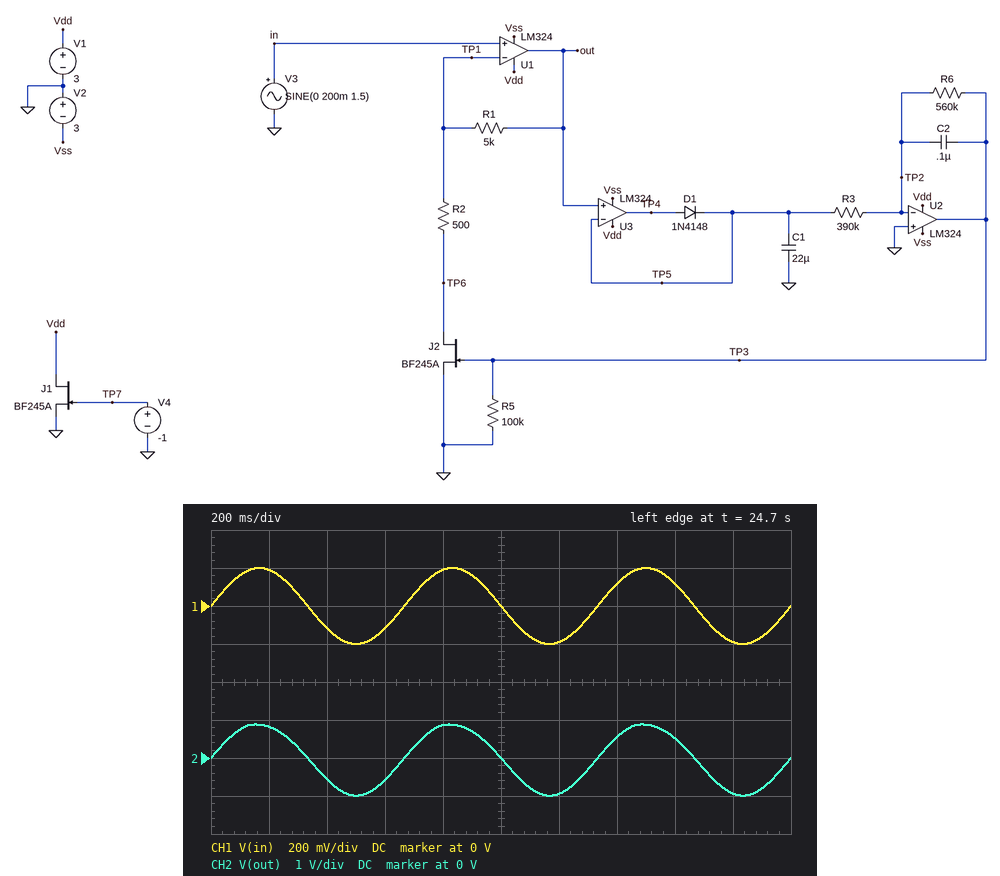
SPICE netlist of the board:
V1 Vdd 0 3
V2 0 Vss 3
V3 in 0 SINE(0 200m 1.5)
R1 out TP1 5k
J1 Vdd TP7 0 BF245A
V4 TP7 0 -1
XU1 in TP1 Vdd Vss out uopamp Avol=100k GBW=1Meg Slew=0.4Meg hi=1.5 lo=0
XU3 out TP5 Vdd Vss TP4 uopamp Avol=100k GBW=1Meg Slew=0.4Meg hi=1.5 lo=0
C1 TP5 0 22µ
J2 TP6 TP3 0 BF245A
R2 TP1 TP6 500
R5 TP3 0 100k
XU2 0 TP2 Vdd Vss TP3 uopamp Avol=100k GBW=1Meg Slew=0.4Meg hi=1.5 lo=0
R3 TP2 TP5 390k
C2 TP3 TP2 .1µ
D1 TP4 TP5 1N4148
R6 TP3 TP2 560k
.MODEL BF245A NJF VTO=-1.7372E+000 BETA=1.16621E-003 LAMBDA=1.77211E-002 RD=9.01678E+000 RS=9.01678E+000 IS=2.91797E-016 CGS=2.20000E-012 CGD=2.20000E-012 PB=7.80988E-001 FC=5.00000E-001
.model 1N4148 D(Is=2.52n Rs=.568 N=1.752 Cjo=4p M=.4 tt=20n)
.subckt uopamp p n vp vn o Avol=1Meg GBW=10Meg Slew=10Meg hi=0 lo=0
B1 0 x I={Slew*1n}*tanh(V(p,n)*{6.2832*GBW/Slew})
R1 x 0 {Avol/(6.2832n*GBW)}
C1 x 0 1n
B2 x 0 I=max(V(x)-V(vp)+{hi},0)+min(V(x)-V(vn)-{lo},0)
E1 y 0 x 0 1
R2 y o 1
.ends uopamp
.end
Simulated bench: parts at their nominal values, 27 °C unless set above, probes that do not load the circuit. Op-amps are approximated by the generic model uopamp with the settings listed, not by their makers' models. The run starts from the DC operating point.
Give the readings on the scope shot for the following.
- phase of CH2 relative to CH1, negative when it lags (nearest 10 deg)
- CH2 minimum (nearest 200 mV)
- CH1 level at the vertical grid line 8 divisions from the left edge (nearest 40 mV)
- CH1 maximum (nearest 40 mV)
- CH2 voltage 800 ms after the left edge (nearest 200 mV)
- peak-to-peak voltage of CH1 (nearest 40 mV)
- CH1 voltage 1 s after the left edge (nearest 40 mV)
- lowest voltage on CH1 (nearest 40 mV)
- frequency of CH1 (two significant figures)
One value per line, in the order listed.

0 deg
-1.0 V
120 mV
200 mV
800 mV
400 mV
0 V
-200 mV
1.5 Hz
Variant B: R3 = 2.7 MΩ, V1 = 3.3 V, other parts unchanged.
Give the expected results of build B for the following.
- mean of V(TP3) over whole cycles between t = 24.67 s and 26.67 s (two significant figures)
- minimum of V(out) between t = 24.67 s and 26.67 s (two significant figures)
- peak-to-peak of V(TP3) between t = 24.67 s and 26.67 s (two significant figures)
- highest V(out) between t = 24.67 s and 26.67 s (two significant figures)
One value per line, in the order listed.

-290 mV
-1.4 V
2.3 mV
1.4 V
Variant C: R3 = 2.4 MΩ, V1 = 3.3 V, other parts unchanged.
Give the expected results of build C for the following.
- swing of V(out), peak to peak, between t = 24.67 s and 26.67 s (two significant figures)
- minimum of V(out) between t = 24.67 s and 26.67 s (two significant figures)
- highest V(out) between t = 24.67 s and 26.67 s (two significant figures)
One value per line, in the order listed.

2.8 V
-1.4 V
1.4 V
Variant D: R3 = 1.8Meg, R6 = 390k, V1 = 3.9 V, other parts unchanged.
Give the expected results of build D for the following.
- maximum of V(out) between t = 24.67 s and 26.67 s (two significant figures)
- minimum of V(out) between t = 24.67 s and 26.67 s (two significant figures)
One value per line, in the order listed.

1.4 V
-1.4 V
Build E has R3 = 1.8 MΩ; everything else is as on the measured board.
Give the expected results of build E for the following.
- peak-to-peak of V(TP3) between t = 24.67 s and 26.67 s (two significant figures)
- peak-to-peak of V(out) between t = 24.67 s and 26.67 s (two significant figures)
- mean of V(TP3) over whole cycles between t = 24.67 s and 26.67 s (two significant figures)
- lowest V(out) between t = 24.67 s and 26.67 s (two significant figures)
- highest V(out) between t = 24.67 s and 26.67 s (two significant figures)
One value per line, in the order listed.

3.8 mV
2.8 V
-360 mV
-1.4 V
1.4 V
